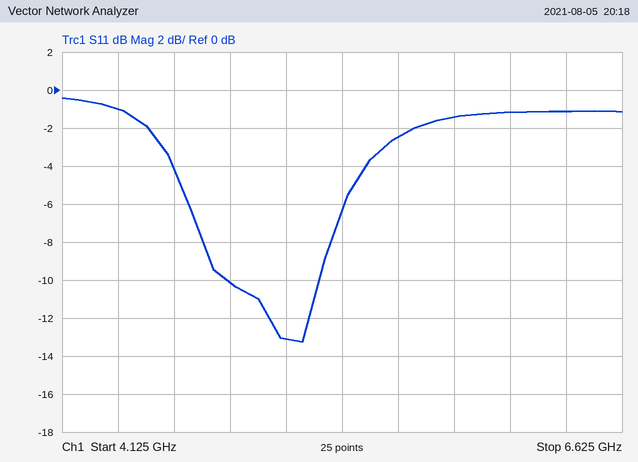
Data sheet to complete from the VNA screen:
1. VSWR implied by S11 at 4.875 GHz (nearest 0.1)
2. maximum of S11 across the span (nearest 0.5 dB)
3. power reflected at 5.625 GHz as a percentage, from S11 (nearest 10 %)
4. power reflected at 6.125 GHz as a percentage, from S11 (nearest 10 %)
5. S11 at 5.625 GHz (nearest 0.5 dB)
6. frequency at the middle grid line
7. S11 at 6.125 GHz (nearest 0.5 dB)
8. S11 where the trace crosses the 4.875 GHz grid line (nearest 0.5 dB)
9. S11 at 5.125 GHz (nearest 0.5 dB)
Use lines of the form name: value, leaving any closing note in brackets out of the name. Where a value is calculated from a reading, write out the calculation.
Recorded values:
VSWR implied by S11 at 4.875 GHz: |Γ| = 10^(-10/20) = 0.3162; VSWR = (1 + 0.3162)/(1 − 0.3162) ≈ 1.9
maximum of S11 across the span: -0.5 dB
power reflected at 5.625 GHz as a percentage, from S11: 10^(-2.5/10) ≈ 56.2 %, so 60 % to the nearest 10 %
power reflected at 6.125 GHz as a percentage, from S11: 10^(-1/10) ≈ 79.4 %, so 80 % to the nearest 10 %
S11 at 5.625 GHz: -2.5 dB
frequency at the middle grid line: 5.375 GHz
S11 at 6.125 GHz: -1.0 dB
S11 where the trace crosses the 4.875 GHz grid line: -10.0 dB
S11 at 5.125 GHz: -13.0 dB
